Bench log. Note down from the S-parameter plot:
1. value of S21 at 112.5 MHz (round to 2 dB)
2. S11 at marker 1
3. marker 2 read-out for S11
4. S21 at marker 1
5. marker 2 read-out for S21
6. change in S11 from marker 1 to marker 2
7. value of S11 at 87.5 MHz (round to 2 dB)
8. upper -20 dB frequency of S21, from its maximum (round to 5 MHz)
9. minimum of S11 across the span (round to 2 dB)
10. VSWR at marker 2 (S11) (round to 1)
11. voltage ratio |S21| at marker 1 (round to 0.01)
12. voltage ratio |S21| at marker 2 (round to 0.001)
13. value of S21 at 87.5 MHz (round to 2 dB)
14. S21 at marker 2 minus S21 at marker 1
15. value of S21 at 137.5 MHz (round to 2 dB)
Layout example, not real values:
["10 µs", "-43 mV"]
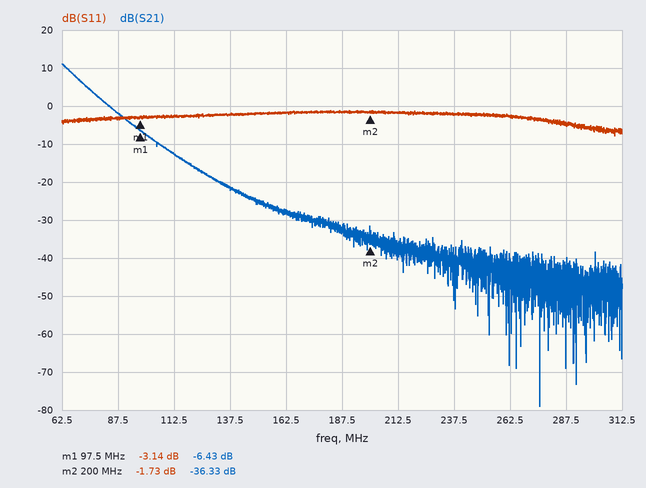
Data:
["-12 dB", "-3.14 dB", "-1.73 dB", "-6.43 dB", "-36.33 dB", "1.41 dB", "-4 dB", "105 MHz", "-8 dB", "10", "0.48", "0.015", "-2 dB", "-29.90 dB", "-22 dB"]
